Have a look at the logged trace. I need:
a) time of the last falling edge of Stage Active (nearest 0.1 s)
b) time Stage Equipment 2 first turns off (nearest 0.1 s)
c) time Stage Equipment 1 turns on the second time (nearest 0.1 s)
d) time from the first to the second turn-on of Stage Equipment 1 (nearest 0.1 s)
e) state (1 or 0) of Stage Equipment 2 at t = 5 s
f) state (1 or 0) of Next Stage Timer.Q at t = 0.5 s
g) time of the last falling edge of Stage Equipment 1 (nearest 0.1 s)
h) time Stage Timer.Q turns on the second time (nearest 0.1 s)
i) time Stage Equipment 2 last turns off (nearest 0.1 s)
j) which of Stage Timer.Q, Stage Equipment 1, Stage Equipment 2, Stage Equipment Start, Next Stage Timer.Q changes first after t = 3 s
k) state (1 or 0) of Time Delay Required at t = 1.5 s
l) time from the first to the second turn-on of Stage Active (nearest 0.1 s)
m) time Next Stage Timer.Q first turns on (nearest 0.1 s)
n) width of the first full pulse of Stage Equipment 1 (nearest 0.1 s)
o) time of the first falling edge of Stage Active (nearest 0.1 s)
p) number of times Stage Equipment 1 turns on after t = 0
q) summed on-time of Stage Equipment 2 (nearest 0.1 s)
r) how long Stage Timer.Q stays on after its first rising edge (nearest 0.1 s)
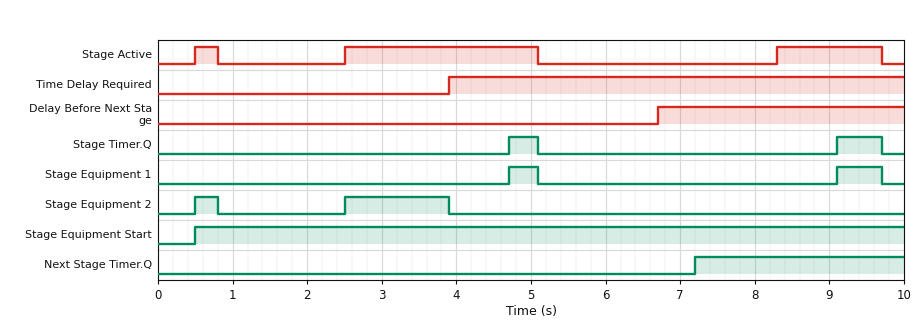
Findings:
9.7 s
0.8 s
9.1 s
4.4 s
0
0
9.7 s
9.1 s
3.9 s
Stage Equipment 2
0
2.0 s
7.2 s
0.4 s
0.8 s
2
1.7 s
0.4 s
